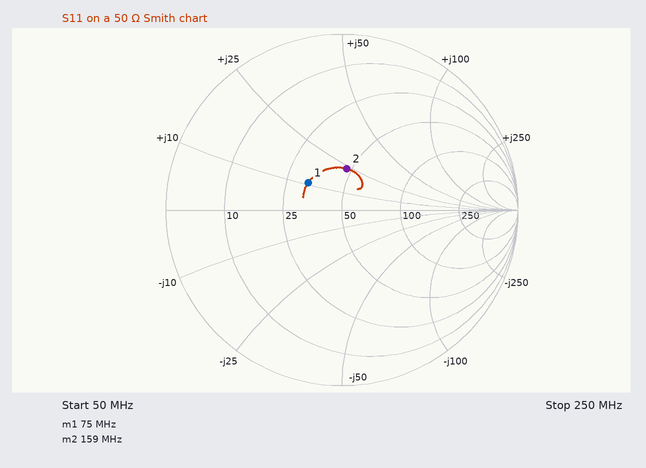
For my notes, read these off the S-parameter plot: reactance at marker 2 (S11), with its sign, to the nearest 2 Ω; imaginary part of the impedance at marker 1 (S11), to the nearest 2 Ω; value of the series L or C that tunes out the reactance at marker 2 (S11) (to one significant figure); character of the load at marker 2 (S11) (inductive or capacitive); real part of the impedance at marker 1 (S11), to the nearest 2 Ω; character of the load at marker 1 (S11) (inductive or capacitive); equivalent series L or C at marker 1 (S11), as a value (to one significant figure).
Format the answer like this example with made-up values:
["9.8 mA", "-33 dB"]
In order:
["+24 Ω", "+10 Ω", "40 pF", "inductive", "32 Ω", "inductive", "20 nH"]
